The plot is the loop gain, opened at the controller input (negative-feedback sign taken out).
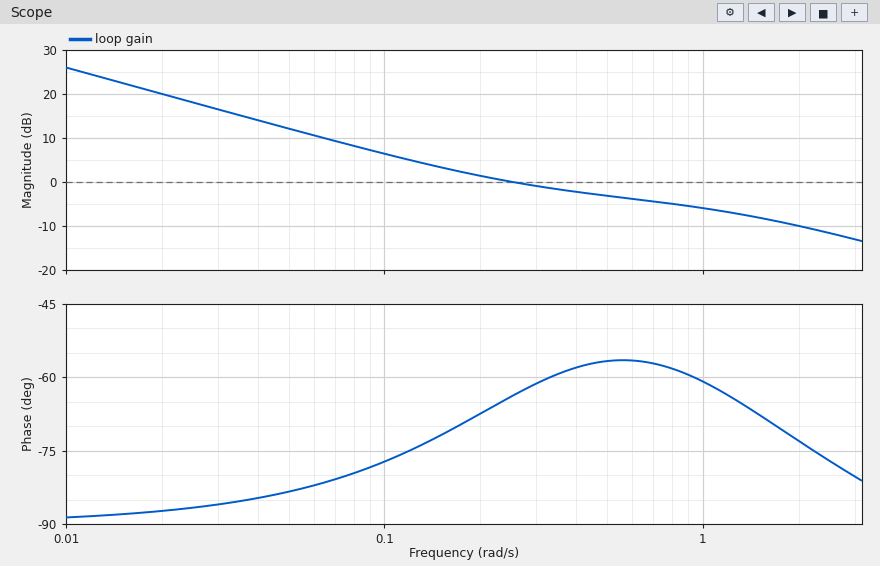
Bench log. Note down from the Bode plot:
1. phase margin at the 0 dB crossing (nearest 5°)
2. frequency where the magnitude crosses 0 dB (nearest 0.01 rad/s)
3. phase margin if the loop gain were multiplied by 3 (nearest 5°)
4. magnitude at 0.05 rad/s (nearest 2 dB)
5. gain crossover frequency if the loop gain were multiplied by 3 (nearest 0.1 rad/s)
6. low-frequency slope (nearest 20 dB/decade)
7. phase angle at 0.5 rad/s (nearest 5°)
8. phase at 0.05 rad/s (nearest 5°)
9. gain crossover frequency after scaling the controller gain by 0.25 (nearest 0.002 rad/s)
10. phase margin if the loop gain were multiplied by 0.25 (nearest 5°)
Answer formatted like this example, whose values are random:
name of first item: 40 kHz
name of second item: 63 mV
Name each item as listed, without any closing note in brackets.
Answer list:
phase margin at the 0 dB crossing: 115°
frequency where the magnitude crosses 0 dB: 0.25 rad/s
phase margin if the loop gain were multiplied by 3: 110°
magnitude at 0.05 rad/s: 12 dB
gain crossover frequency if the loop gain were multiplied by 3: 1.9 rad/s
low-frequency slope: -20 dB/decade
phase angle at 0.5 rad/s: -55°
phase at 0.05 rad/s: -85°
gain crossover frequency after scaling the controller gain by 0.25: 0.050 rad/s
phase margin if the loop gain were multiplied by 0.25: 95°
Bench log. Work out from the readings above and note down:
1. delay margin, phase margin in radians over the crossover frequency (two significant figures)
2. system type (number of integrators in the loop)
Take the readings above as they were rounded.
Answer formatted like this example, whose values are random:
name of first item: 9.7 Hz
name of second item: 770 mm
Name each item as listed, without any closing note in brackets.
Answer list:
delay margin, phase margin in radians over the crossover frequency: 8.0 s
system type: 1
